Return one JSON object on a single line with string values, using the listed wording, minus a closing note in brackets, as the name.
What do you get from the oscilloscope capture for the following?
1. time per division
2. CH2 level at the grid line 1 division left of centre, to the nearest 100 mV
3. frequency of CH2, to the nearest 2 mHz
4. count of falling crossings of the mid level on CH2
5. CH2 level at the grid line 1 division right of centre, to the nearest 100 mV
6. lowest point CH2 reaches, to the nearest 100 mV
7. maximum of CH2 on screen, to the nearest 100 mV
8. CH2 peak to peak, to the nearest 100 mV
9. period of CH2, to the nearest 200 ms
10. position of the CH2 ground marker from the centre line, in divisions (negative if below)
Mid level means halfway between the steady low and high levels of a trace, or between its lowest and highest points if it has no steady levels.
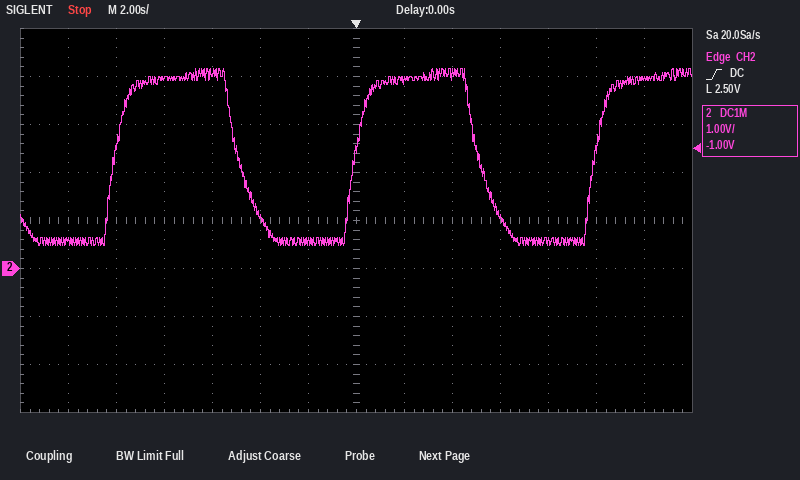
{"time per division": "2 s", "CH2 level at the grid line 1 division left of centre, to the nearest 100 mV": "600 mV", "frequency of CH2, to the nearest 2 mHz": "100 mHz", "count of falling crossings of the mid level on CH2": "2", "CH2 level at the grid line 1 division right of centre, to the nearest 100 mV": "3.9 V", "lowest point CH2 reaches, to the nearest 100 mV": "500 mV", "maximum of CH2 on screen, to the nearest 100 mV": "4.2 V", "CH2 peak to peak, to the nearest 100 mV": "3.7 V", "period of CH2, to the nearest 200 ms": "10.0 s", "position of the CH2 ground marker from the centre line, in divisions": "-1.0 div"}
